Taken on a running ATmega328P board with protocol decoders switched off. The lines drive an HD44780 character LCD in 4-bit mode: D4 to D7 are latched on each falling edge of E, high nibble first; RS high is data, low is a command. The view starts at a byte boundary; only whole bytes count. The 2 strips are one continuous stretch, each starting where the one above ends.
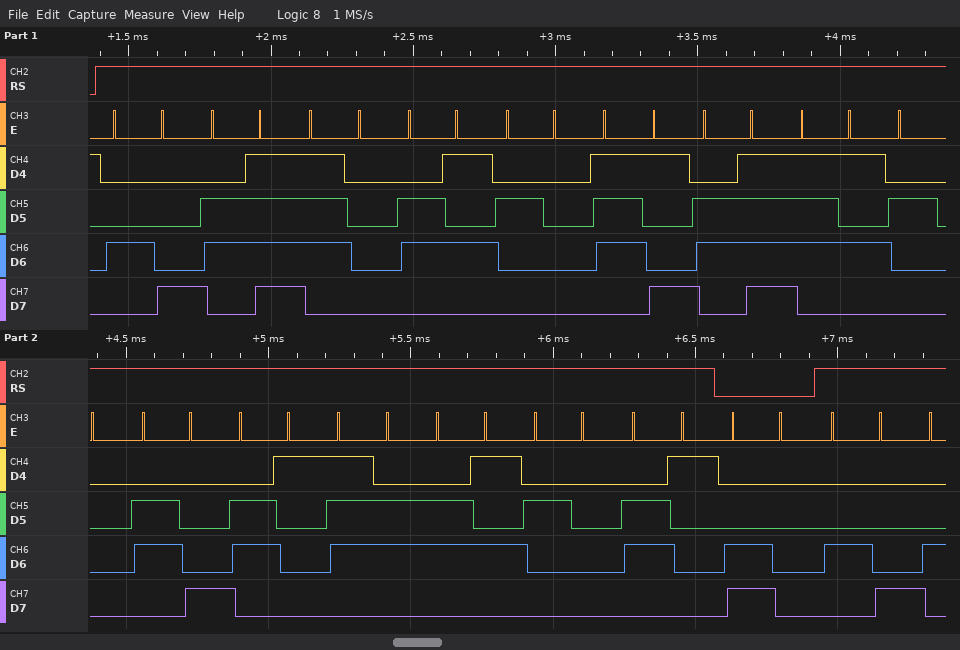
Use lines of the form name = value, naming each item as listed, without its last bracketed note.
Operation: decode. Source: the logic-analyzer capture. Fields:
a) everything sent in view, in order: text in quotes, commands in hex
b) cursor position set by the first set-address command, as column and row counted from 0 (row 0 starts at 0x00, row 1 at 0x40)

everything sent in view, in order: text in quotes, commands in hex = "Hope you have a" 0xC0 "H"
cursor position set by the first set-address command, as column and row counted from 0 = column 0, row 1
